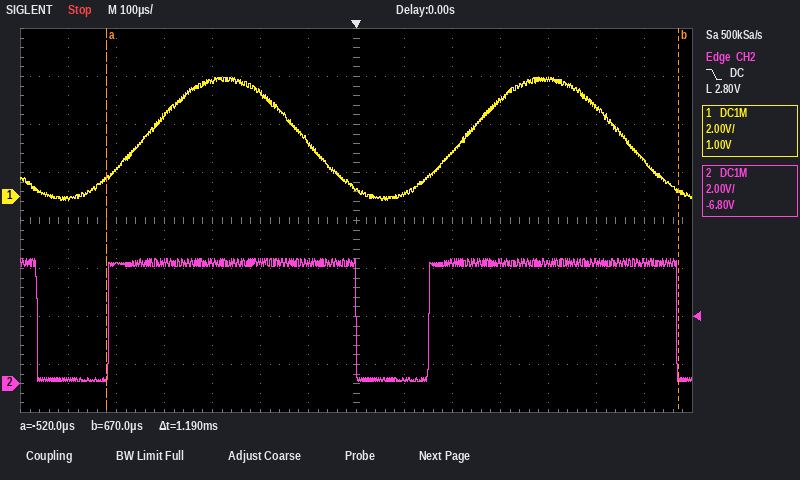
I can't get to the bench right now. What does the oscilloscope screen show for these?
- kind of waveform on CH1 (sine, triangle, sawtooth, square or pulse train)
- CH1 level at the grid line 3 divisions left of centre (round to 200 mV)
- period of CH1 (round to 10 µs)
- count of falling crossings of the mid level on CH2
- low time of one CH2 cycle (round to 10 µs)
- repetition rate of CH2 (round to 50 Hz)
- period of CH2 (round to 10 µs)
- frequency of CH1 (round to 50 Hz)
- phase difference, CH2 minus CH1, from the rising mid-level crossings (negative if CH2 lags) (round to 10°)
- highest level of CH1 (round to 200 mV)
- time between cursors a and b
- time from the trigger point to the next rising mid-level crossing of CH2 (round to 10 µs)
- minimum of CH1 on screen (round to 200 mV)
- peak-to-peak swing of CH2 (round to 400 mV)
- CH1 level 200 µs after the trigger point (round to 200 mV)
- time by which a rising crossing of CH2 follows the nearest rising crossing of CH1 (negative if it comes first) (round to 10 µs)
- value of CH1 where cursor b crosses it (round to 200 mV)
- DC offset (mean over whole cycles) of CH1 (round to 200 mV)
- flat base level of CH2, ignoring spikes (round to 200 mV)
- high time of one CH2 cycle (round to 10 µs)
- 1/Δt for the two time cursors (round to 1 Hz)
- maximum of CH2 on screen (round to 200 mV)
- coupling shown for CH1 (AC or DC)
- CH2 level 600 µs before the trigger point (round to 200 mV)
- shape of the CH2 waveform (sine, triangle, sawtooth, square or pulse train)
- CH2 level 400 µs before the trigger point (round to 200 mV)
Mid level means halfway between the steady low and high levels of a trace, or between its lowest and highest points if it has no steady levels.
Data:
sine
4.8 V
670 µs
3
150 µs
1.50 kHz
670 µs
1.50 kHz
+40°
5.0 V
1.19 ms
150 µs
-200 mV
5.2 V
1.8 V
-70 µs
200 mV
2.4 V
200 mV
520 µs
840 Hz
5.2 V
DC
200 mV
pulse train
5.0 V
